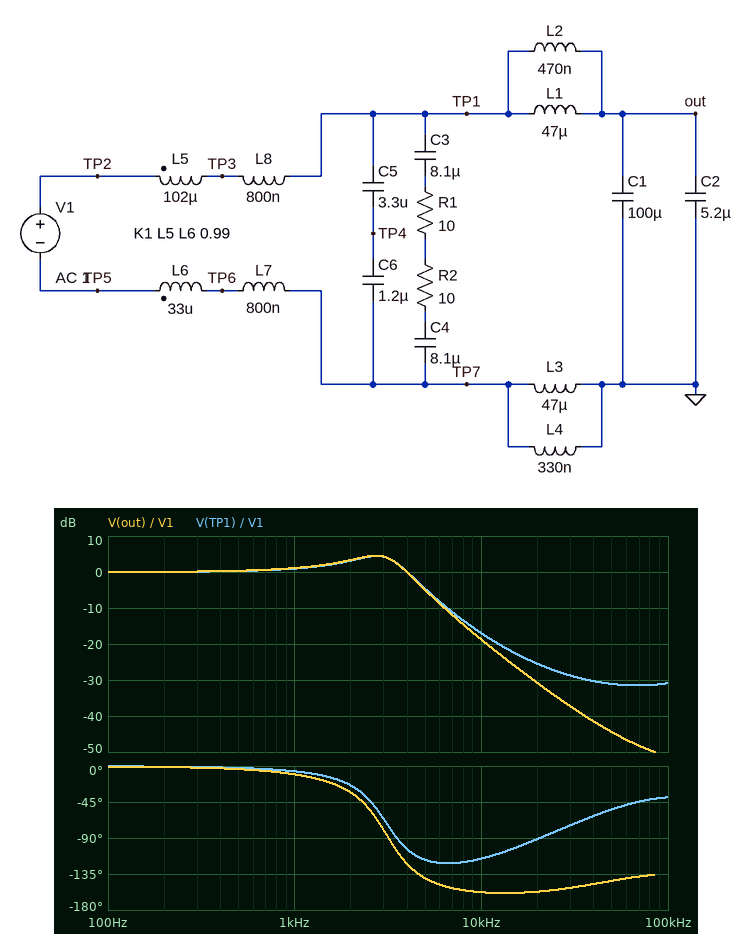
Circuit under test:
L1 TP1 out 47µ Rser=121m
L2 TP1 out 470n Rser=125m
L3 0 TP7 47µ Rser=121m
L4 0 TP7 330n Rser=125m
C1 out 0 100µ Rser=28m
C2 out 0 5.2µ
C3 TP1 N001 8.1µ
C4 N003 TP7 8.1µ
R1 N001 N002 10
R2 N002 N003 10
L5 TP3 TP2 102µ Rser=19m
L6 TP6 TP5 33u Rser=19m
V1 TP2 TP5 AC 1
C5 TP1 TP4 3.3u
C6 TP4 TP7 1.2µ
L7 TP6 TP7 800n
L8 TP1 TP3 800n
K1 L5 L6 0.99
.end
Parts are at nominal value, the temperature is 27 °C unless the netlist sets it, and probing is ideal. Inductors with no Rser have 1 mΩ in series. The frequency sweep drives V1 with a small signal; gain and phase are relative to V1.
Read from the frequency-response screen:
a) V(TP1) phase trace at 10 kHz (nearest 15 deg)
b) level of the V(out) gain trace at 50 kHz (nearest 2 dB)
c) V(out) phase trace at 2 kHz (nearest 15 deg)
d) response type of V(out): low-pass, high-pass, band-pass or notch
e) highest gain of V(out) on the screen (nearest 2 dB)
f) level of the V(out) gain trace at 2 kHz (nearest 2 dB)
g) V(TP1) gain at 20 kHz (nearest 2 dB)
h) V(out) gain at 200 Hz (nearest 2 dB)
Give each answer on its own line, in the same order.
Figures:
-120 deg
-44 dB
-30 deg
low-pass
4 dB
4 dB
-26 dB
0 dB
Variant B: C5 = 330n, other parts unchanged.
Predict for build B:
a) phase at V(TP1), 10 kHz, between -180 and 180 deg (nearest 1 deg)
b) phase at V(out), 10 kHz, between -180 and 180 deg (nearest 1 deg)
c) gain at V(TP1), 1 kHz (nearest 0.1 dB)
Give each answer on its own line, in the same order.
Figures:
-115 deg
-157 deg
0.9 dB
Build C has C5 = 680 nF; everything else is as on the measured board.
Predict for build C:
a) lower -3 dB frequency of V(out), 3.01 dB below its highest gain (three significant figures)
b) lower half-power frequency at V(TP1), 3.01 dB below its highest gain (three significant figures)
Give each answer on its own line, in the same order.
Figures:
1.22 kHz
1.26 kHz
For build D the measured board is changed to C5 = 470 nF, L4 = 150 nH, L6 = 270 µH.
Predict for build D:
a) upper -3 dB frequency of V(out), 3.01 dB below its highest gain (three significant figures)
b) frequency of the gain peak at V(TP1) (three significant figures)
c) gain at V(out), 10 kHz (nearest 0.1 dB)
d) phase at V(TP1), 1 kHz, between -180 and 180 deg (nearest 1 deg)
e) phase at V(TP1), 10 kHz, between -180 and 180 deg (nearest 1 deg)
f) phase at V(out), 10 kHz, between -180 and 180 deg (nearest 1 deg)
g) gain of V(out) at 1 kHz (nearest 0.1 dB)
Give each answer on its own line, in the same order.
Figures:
2.54 kHz
2.07 kHz
-25.2 dB
-8 deg
-122 deg
-164 deg
2.1 dB
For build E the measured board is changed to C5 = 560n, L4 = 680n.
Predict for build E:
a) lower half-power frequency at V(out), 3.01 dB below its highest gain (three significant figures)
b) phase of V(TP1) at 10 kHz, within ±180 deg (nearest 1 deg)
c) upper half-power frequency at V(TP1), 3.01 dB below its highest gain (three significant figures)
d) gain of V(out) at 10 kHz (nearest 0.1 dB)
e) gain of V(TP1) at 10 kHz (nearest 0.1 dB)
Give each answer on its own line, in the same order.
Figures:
1.26 kHz
-116 deg
3.70 kHz
-18.9 dB
-17.1 dB
